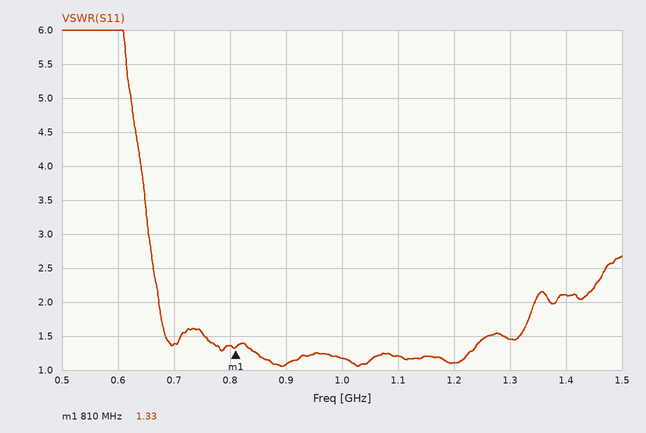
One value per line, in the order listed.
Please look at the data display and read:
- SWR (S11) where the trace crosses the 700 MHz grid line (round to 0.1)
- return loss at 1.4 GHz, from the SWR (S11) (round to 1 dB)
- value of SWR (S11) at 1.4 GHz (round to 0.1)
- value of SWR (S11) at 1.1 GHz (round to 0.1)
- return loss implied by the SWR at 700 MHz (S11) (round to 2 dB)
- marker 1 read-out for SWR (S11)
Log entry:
1.4
9 dB
2.1
1.2
16 dB
1.33
